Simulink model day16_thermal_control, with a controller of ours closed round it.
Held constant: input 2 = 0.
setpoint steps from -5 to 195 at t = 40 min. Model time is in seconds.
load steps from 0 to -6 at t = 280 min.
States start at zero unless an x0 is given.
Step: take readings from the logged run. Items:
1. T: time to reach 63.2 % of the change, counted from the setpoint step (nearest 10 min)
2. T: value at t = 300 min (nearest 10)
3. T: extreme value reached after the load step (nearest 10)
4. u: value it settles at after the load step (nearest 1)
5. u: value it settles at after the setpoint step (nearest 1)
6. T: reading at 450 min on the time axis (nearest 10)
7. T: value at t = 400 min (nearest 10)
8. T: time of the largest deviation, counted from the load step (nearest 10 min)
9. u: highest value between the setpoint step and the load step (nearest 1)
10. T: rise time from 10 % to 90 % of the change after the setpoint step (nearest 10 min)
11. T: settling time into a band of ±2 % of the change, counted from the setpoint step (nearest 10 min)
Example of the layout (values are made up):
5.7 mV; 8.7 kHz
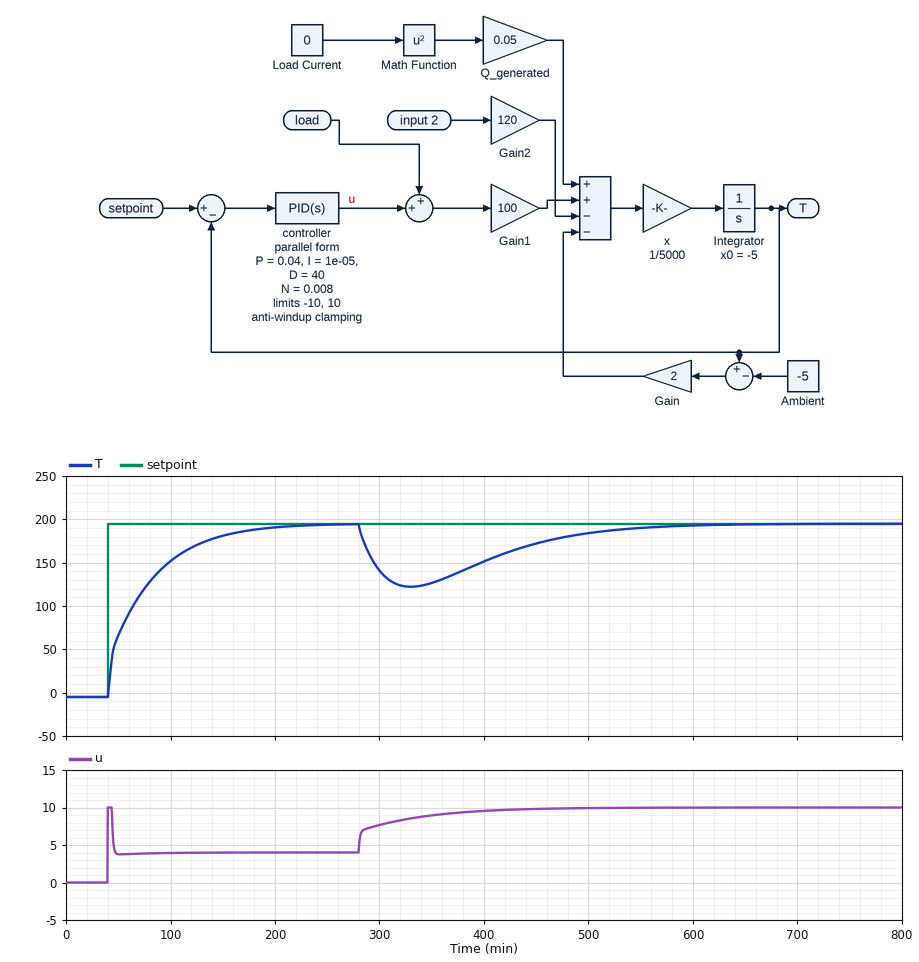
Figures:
40 min; 140; 120; 10; 4; 170; 150; 50 min; 10; 90 min; 160 min
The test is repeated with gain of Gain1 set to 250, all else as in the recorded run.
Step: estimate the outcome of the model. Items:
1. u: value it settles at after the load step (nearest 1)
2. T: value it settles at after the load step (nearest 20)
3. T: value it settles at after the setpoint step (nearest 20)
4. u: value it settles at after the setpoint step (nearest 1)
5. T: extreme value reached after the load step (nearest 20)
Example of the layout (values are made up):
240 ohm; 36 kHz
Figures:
8; 200; 200; 2; 100
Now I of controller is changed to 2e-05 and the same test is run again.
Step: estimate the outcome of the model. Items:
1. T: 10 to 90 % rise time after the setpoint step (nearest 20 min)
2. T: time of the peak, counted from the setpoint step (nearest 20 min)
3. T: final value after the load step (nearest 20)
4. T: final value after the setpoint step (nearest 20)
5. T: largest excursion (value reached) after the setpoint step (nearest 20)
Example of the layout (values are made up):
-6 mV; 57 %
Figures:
60 min; 120 min; 200; 200; 200
